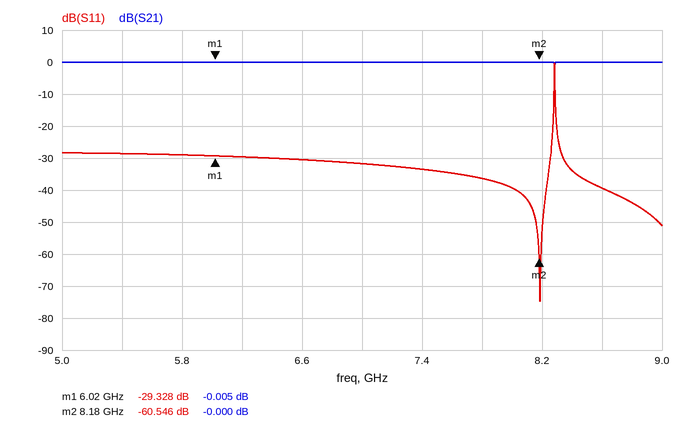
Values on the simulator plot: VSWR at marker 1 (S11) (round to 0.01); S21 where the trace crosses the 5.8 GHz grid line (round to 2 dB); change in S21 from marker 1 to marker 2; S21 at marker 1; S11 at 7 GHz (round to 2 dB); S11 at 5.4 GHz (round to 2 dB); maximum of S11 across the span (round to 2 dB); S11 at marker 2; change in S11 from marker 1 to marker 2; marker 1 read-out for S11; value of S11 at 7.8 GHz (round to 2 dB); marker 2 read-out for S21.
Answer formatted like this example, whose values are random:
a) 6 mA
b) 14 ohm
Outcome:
a) 1.07
b) 0 dB
c) 0.005 dB
d) -0.005 dB
e) -32 dB
f) -28 dB
g) 0 dB
h) -60.546 dB
i) -31.218 dB
j) -29.328 dB
k) -36 dB
l) -0.000 dB
